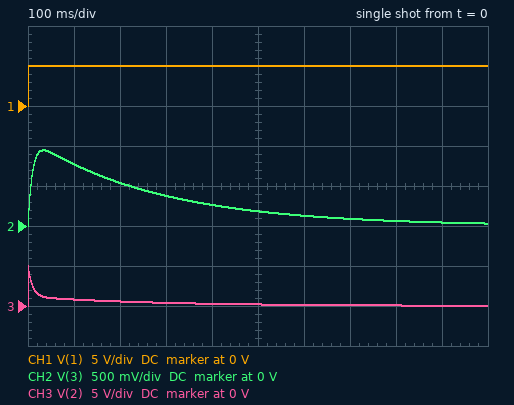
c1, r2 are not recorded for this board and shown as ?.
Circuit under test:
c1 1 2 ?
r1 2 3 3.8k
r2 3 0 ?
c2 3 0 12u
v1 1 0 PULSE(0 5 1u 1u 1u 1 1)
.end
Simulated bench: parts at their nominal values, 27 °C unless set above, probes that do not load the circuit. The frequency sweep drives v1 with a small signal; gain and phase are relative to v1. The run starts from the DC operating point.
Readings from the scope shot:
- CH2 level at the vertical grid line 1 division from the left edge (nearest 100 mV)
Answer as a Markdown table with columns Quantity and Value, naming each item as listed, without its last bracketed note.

| Quantity | Value |
|---|---|
| CH2 level at the vertical grid line 1 division from the left edge | 800 mV |
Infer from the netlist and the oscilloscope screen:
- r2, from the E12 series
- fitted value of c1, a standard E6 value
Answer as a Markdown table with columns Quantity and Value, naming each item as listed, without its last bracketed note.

| Quantity | Value |
|---|---|
| r2, from the E12 series | 18 kΩ |
| fitted value of c1, a standard E6 value | 3.3 µF |
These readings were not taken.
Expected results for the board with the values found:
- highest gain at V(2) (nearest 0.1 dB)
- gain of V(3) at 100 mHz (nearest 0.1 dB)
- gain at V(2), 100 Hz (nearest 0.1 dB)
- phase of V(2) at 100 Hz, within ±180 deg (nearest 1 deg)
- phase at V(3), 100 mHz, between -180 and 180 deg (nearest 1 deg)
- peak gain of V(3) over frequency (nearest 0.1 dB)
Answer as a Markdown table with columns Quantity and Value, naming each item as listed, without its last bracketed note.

| Quantity | Value |
|---|---|
| highest gain at V(2) | 0 dB |
| gain of V(3) at 100 mHz | -28.7 dB |
| gain at V(2), 100 Hz | -0.1 dB |
| phase of V(2) at 100 Hz, within ±180 deg | 7 deg |
| phase at V(3), 100 mHz, between -180 and 180 deg | 80 deg |
| peak gain of V(3) over frequency | -13.7 dB |
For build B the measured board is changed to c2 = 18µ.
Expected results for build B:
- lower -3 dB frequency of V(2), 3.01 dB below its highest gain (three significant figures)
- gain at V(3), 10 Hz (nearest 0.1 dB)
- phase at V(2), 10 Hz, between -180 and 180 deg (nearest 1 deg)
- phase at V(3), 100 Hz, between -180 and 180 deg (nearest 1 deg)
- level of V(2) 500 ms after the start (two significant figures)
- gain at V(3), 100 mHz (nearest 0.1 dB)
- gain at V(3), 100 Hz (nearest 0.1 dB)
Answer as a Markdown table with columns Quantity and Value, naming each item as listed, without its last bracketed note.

| Quantity | Value |
|---|---|
| lower -3 dB frequency of V(2), 3.01 dB below its highest gain | 14.6 Hz |
| gain at V(3), 10 Hz | -17.8 dB |
| phase at V(2), 10 Hz, between -180 and 180 deg | 43 deg |
| phase at V(3), 100 Hz, between -180 and 180 deg | -81 deg |
| level of V(2) 500 ms after the start | 220 mV |
| gain at V(3), 100 mHz | -28.8 dB |
| gain at V(3), 100 Hz | -32.8 dB |
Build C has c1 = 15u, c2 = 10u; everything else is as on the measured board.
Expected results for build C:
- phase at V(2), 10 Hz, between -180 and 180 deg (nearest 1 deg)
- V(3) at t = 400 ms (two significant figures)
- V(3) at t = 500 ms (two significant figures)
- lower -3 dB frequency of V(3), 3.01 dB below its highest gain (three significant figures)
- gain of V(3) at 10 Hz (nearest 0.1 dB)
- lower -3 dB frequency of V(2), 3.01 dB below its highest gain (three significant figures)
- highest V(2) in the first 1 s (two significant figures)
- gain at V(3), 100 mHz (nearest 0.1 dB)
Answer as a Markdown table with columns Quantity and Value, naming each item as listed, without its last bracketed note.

| Quantity | Value |
|---|---|
| phase at V(2), 10 Hz, between -180 and 180 deg | 12 deg |
| V(3) at t = 400 ms | 1.3 V |
| V(3) at t = 500 ms | 1.0 V |
| lower -3 dB frequency of V(3), 3.01 dB below its highest gain | 302 mHz |
| gain of V(3) at 10 Hz | -9.5 dB |
| lower -3 dB frequency of V(2), 3.01 dB below its highest gain | 2.53 Hz |
| highest V(2) in the first 1 s | 5.0 V |
| gain at V(3), 100 mHz | -15.8 dB |
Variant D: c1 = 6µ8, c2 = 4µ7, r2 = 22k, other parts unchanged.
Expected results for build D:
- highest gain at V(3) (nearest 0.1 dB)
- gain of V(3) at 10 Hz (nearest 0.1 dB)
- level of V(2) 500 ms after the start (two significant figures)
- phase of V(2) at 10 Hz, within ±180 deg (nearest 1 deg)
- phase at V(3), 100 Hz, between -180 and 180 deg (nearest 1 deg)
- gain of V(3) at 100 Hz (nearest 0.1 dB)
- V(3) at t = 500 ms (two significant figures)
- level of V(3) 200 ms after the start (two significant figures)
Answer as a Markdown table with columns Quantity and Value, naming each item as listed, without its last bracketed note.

| Quantity | Value |
|---|---|
| highest gain at V(3) | -5.4 dB |
| gain of V(3) at 10 Hz | -6.5 dB |
| level of V(2) 500 ms after the start | 500 mV |
| phase of V(2) at 10 Hz, within ±180 deg | 15 deg |
| phase at V(3), 100 Hz, between -180 and 180 deg | -81 deg |
| gain of V(3) at 100 Hz | -21.1 dB |
| V(3) at t = 500 ms | 450 mV |
| level of V(3) 200 ms after the start | 1.4 V |
